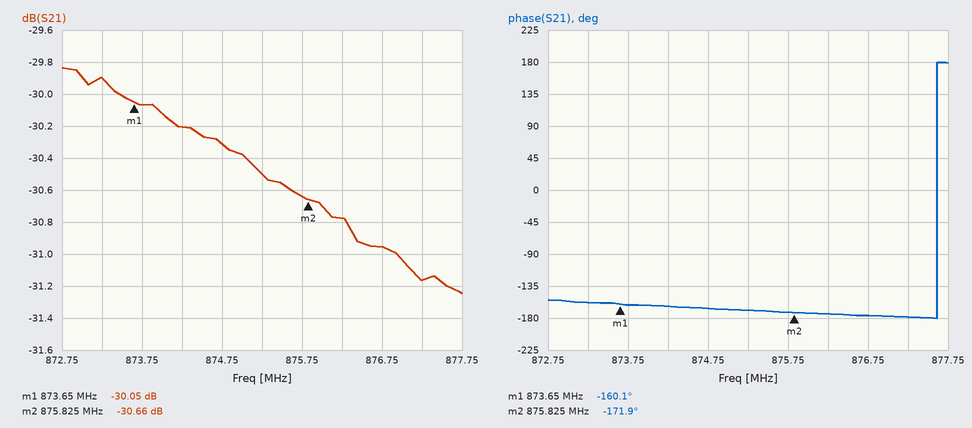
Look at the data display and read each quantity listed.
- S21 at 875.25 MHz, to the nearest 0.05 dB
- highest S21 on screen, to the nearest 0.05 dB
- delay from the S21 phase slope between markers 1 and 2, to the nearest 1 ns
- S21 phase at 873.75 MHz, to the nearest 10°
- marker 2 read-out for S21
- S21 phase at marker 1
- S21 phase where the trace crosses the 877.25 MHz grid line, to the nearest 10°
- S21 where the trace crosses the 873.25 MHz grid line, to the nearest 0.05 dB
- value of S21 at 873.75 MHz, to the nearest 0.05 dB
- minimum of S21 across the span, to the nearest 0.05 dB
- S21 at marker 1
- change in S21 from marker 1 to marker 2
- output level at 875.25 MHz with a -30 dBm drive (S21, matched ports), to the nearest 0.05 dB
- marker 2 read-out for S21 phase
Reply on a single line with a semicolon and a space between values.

-30.50 dB; -29.85 dB; 15 ns; -160°; -30.66 dB; -160.1°; -180°; -29.90 dB; -30.05 dB; -31.25 dB; -30.05 dB; -0.61 dB; -60.50 dBm; -171.9°
